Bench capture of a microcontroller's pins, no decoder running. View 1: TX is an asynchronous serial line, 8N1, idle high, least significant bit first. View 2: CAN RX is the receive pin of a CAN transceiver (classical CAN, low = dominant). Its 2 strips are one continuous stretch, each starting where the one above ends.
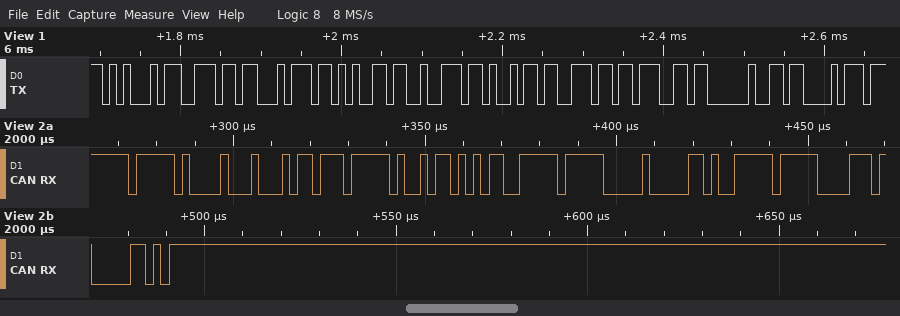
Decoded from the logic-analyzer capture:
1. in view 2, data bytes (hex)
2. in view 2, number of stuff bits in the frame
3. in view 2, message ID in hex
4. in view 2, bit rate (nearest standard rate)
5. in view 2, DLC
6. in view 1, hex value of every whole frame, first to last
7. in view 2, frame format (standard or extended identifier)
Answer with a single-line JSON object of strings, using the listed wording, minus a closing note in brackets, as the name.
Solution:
{"in view 2, data bytes": "B7 7E 5A B3 FF 00 53 FF", "in view 2, number of stuff bits in the frame": "9", "in view 2, message ID in hex": "0x7E1", "in view 2, bit rate": "500 kbit/s", "in view 2, DLC": "8", "in view 1, hex value of every whole frame, first to last": "45 6E 74 65 72 69 6E 67 20 43", "in view 2, frame format": "standard"}
